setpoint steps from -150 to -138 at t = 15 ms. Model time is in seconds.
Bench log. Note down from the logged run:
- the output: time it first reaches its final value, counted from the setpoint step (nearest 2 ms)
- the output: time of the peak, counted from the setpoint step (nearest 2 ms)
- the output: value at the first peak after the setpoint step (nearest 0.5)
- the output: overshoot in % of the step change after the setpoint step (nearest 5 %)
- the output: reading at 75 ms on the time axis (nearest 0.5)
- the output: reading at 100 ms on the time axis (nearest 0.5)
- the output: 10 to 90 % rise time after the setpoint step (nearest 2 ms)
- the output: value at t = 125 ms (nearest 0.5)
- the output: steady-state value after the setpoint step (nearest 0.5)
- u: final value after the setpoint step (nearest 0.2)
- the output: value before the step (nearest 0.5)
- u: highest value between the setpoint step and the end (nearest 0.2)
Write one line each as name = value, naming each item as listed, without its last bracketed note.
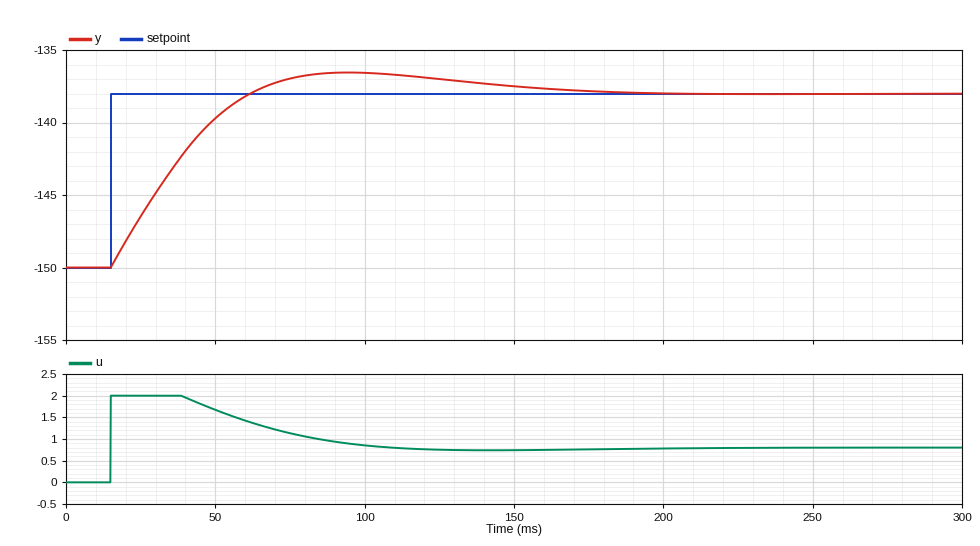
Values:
the output: time it first reaches its final value, counted from the setpoint step = 46 ms
the output: time of the peak, counted from the setpoint step = 80 ms
the output: value at the first peak after the setpoint step = -136.5
the output: overshoot in % of the step change after the setpoint step = 10 %
the output: reading at 75 ms on the time axis = -137.0
the output: reading at 100 ms on the time axis = -136.5
the output: 10 to 90 % rise time after the setpoint step = 34 ms
the output: value at t = 125 ms = -137.0
the output: steady-state value after the setpoint step = -138.0
u: final value after the setpoint step = 0.8
the output: value before the step = -150.0
u: highest value between the setpoint step and the end = 2.0
